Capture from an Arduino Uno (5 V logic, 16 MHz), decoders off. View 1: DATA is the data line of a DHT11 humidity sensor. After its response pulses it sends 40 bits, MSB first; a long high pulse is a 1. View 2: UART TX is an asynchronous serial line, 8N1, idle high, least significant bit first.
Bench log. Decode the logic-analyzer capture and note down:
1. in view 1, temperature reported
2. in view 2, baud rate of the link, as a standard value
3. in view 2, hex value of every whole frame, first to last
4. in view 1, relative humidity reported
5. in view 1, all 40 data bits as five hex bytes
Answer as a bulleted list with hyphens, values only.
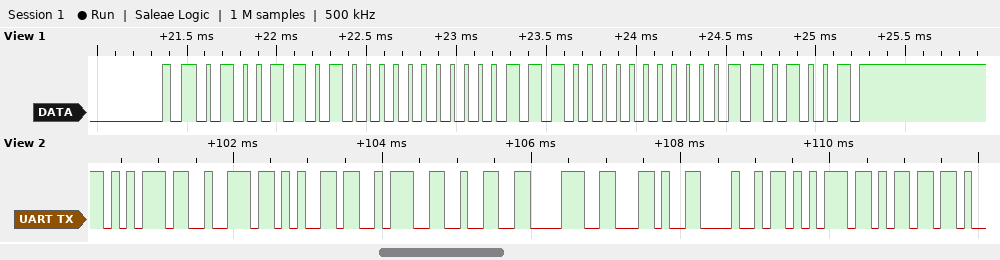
- 28.0 °C
- 9600 baud
- 0x75 0x72 0x65 0x3A 0x32 0x38 0x2C 0x48 0x75 0x6D
- 77 %
- 4D 00 1C 00 69
